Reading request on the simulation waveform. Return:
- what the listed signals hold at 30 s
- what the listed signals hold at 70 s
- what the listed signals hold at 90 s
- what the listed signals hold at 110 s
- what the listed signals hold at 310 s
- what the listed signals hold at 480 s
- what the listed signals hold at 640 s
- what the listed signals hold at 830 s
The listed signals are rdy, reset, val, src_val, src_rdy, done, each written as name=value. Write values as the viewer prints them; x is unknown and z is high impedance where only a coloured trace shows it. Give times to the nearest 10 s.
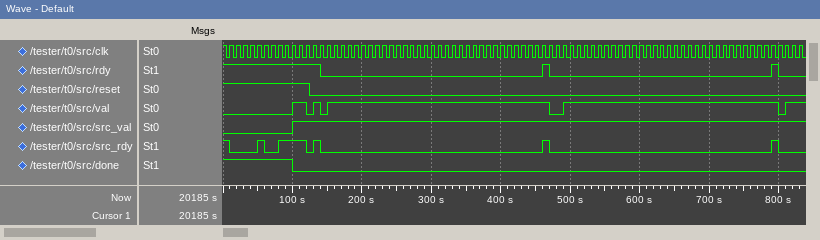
rdy=1, reset=1, val=0, src_val=0, src_rdy=0, done=1
rdy=1, reset=1, val=0, src_val=0, src_rdy=0, done=1
rdy=1, reset=1, val=0, src_val=0, src_rdy=1, done=1
rdy=1, reset=1, val=1, src_val=1, src_rdy=1, done=0
rdy=0, reset=0, val=1, src_val=1, src_rdy=0, done=0
rdy=0, reset=0, val=0, src_val=1, src_rdy=0, done=0
rdy=0, reset=0, val=1, src_val=1, src_rdy=0, done=0
rdy=0, reset=0, val=1, src_val=1, src_rdy=0, done=0
